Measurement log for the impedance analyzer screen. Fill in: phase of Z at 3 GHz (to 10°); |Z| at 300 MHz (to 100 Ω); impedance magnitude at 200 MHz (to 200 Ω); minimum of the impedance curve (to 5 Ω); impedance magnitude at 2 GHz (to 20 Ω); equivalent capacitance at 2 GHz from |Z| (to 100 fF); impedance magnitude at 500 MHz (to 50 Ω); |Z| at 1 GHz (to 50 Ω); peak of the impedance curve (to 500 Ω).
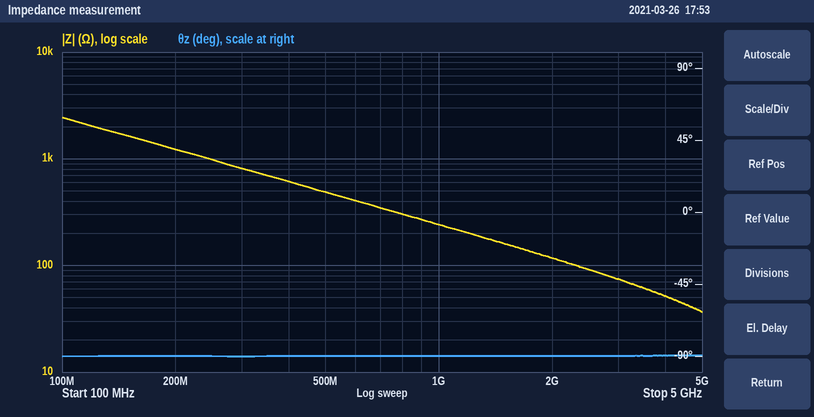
-90°
800 Ω
1.2 kΩ
35 Ω
120 Ω
700 fF
500 Ω
250 Ω
2.5 kΩ
